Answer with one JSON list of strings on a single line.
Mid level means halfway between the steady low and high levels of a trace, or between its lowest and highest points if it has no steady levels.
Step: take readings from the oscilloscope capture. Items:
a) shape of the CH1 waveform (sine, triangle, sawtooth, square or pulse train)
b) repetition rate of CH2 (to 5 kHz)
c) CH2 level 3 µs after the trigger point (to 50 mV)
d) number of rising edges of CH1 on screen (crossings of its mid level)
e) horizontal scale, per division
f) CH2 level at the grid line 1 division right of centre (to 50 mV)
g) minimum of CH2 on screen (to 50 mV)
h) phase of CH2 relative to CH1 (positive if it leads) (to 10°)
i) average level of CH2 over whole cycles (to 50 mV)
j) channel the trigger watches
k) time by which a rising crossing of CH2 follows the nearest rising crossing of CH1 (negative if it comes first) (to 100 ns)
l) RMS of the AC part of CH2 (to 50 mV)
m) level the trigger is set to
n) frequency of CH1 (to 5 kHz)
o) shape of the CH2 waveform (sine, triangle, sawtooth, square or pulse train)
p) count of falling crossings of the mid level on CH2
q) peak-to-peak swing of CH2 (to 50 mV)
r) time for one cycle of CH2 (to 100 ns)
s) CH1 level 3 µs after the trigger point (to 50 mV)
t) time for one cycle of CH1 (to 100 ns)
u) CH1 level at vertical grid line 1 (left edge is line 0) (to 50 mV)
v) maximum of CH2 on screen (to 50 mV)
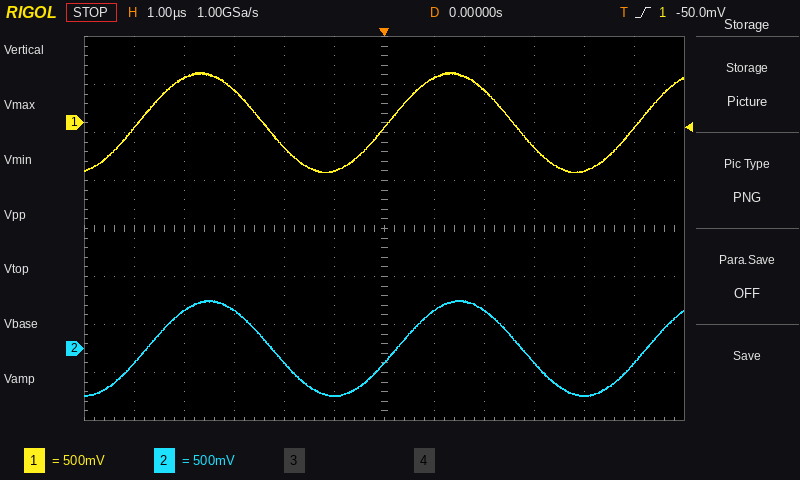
["sine", "200 kHz", "-150 mV", "3", "1 µs", "400 mV", "-500 mV", "-10°", "0 mV", "CH1", "+200 ns", "350 mV", "-50.0 mV", "200 kHz", "sine", "2", "1.00 V", "5.0 µs", "-250 mV", "5.0 µs", "-50 mV", "500 mV"]
